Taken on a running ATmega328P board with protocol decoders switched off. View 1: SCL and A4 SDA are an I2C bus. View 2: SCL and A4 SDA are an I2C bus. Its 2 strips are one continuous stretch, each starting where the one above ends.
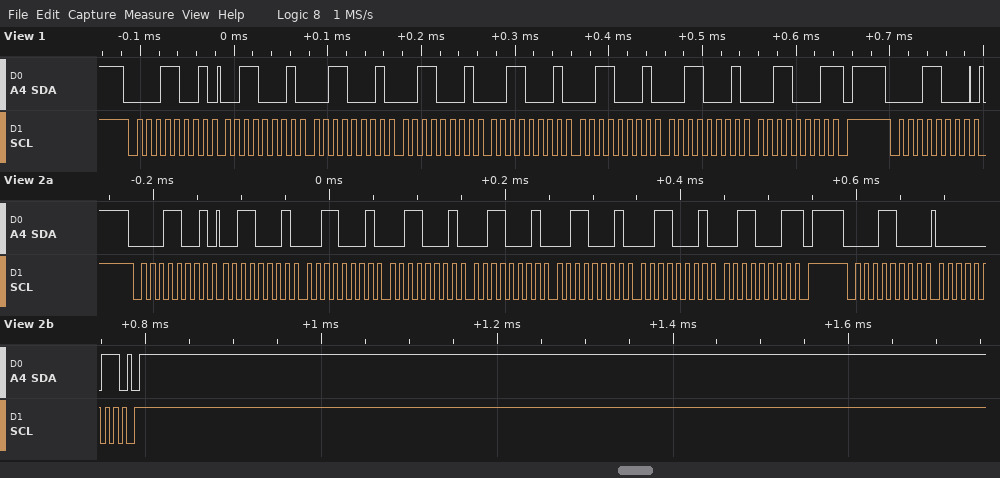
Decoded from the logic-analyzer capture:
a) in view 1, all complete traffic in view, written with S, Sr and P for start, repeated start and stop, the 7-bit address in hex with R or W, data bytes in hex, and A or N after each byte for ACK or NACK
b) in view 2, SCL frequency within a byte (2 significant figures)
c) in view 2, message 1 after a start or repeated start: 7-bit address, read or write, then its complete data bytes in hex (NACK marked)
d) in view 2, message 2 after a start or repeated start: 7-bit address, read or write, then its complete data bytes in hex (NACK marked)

S 0CR A 31 A 31 A 31 A 31 A 31 A 31 A 31 N P S 0CW A
100 kHz
0x0C read: 31 31 31 31 31 31 31 NACK
0x0C write: 03
